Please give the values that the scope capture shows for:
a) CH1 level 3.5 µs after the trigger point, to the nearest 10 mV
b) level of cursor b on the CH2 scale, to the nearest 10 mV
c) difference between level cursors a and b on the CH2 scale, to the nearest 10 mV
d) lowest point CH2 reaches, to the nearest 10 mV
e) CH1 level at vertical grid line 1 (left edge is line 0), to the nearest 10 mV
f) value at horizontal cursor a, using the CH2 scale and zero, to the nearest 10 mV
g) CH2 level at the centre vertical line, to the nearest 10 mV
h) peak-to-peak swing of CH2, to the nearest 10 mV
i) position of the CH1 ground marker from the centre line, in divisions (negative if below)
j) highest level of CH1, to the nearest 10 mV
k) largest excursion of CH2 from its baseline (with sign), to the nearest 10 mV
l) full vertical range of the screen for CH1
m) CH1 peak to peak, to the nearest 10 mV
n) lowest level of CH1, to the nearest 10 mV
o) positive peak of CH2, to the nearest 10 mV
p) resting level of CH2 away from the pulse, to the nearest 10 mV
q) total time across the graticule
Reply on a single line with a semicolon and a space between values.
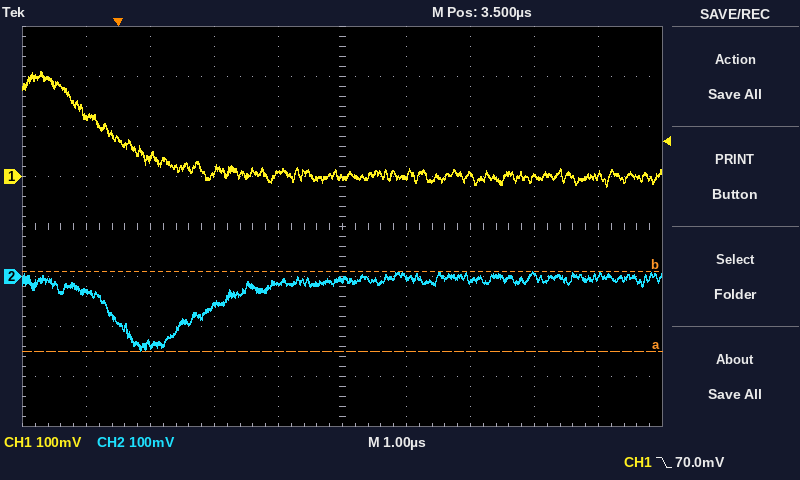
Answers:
0 mV; 10 mV; 160 mV; -150 mV; 120 mV; -150 mV; -10 mV; 160 mV; +1.0 div; 210 mV; -140 mV; 800 mV; 230 mV; -20 mV; 10 mV; -10 mV; 10 µs
